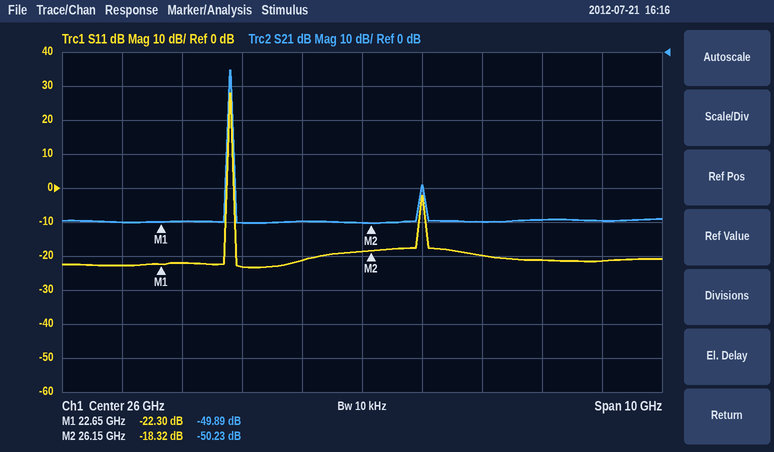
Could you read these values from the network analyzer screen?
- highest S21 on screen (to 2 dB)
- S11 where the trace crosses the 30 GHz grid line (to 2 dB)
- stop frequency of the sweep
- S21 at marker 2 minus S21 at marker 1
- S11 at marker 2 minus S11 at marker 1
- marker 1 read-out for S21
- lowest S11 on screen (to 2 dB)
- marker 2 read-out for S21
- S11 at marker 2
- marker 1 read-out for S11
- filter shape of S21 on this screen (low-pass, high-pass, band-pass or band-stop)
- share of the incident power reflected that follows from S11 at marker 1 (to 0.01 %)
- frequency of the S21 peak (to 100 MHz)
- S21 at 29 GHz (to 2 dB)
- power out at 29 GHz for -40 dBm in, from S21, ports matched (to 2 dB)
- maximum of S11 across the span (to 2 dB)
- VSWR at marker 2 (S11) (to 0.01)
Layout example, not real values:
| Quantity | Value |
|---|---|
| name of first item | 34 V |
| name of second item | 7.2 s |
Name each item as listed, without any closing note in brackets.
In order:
| Quantity | Value |
|---|---|
| highest S21 on screen | -6 dB |
| S11 where the trace crosses the 30 GHz grid line | -22 dB |
| stop frequency of the sweep | 31 GHz |
| S21 at marker 2 minus S21 at marker 1 | -0.34 dB |
| S11 at marker 2 minus S11 at marker 1 | 3.98 dB |
| marker 1 read-out for S21 | -49.89 dB |
| lowest S11 on screen | -24 dB |
| marker 2 read-out for S21 | -50.23 dB |
| S11 at marker 2 | -18.32 dB |
| marker 1 read-out for S11 | -22.30 dB |
| filter shape of S21 on this screen | band-pass |
| share of the incident power reflected that follows from S11 at marker 1 | 0.59 % |
| frequency of the S21 peak | 23.8 GHz |
| S21 at 29 GHz | -50 dB |
| power out at 29 GHz for -40 dBm in, from S21, ports matched | -90 dBm |
| maximum of S11 across the span | 28 dB |
| VSWR at marker 2 (S11) | 1.28 |
